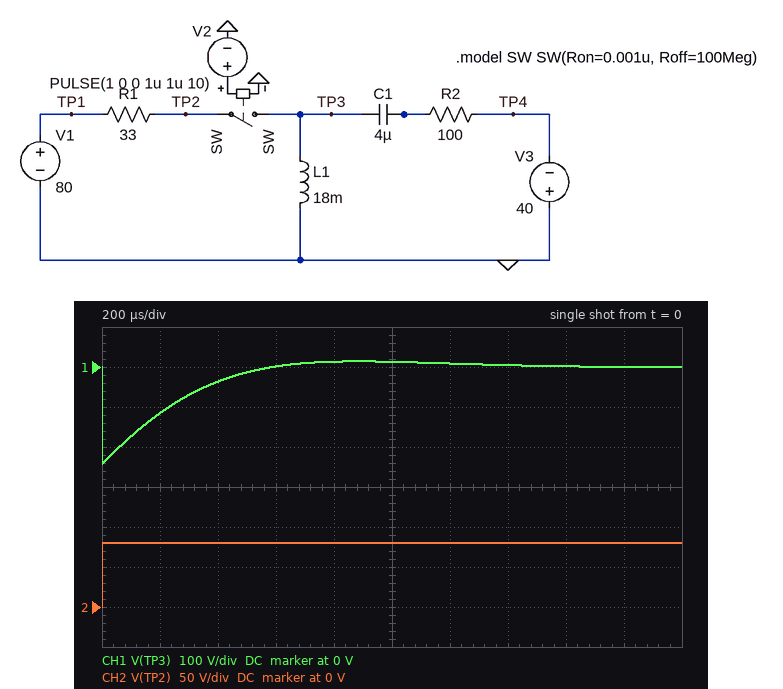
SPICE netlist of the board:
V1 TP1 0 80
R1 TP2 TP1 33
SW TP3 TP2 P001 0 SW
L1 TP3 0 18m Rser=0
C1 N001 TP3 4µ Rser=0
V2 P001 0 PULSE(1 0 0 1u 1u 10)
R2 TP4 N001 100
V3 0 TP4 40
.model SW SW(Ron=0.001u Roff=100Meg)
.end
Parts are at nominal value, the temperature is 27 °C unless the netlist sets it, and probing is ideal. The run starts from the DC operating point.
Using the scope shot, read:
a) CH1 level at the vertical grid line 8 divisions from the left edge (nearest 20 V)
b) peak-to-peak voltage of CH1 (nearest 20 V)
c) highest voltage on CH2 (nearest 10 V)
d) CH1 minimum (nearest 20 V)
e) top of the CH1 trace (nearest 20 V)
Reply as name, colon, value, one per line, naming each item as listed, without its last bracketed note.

CH1 level at the vertical grid line 8 divisions from the left edge: 0 V
peak-to-peak voltage of CH1: 260 V
highest voltage on CH2: 80 V
CH1 minimum: -240 V
top of the CH1 trace: 20 V
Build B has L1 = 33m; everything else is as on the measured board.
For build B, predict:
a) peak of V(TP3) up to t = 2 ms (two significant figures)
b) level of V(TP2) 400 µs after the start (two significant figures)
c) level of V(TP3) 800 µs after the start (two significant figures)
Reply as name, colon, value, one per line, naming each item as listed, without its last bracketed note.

peak of V(TP3) up to t = 2 ms: 31 V
level of V(TP2) 400 µs after the start: 80 V
level of V(TP3) 800 µs after the start: -11 V
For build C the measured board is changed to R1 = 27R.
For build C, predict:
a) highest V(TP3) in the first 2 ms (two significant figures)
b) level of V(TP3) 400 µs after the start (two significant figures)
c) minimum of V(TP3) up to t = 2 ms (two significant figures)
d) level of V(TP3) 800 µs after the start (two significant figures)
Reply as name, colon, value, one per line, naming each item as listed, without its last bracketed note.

highest V(TP3) in the first 2 ms: 17 V
level of V(TP3) 400 µs after the start: -44 V
minimum of V(TP3) up to t = 2 ms: -300 V
level of V(TP3) 800 µs after the start: 16 V
